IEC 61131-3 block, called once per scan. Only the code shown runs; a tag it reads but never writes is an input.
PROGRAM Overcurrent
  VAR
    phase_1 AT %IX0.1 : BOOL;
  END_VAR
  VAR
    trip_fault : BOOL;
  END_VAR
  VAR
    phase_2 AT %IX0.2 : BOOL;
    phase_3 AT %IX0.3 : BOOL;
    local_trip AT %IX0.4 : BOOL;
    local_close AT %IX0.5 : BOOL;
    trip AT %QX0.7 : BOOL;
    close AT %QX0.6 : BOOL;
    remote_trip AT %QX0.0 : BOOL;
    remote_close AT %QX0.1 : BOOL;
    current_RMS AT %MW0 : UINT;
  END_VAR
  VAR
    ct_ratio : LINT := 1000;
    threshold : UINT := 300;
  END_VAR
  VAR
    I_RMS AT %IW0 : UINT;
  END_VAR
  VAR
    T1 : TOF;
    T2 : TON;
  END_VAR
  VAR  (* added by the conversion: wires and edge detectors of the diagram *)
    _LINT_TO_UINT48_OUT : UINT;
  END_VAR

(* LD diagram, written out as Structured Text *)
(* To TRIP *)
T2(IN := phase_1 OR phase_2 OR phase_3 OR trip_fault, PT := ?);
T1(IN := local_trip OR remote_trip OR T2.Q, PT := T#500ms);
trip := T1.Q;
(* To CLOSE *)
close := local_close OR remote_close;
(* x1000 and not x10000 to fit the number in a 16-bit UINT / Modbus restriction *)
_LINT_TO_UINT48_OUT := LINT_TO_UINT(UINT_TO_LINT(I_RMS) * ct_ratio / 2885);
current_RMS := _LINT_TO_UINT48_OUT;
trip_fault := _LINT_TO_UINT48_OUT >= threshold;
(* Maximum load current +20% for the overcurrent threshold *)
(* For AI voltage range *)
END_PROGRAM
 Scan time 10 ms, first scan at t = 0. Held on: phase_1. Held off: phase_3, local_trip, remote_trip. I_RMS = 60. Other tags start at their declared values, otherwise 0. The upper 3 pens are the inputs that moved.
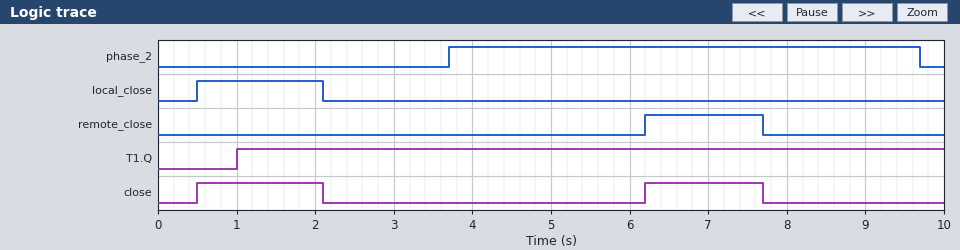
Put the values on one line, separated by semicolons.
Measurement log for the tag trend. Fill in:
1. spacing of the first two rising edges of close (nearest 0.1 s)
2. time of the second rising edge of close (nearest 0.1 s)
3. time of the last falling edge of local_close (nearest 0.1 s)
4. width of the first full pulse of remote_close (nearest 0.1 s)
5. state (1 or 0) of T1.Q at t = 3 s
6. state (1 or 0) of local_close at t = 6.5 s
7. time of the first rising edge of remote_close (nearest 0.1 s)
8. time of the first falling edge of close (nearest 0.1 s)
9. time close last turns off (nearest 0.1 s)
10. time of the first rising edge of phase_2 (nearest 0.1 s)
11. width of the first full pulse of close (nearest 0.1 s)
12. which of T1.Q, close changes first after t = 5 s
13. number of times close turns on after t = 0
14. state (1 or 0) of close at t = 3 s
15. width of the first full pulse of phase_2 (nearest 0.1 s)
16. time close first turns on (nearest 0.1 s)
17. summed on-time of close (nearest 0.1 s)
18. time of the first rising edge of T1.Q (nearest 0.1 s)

5.7 s; 6.2 s; 2.1 s; 1.5 s; 1; 0; 6.2 s; 2.1 s; 7.7 s; 3.7 s; 1.6 s; close; 2; 0; 6.0 s; 0.5 s; 3.1 s; 1.0 s
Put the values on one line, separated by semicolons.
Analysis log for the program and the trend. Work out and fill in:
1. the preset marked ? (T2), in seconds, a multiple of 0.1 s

1.0 s
